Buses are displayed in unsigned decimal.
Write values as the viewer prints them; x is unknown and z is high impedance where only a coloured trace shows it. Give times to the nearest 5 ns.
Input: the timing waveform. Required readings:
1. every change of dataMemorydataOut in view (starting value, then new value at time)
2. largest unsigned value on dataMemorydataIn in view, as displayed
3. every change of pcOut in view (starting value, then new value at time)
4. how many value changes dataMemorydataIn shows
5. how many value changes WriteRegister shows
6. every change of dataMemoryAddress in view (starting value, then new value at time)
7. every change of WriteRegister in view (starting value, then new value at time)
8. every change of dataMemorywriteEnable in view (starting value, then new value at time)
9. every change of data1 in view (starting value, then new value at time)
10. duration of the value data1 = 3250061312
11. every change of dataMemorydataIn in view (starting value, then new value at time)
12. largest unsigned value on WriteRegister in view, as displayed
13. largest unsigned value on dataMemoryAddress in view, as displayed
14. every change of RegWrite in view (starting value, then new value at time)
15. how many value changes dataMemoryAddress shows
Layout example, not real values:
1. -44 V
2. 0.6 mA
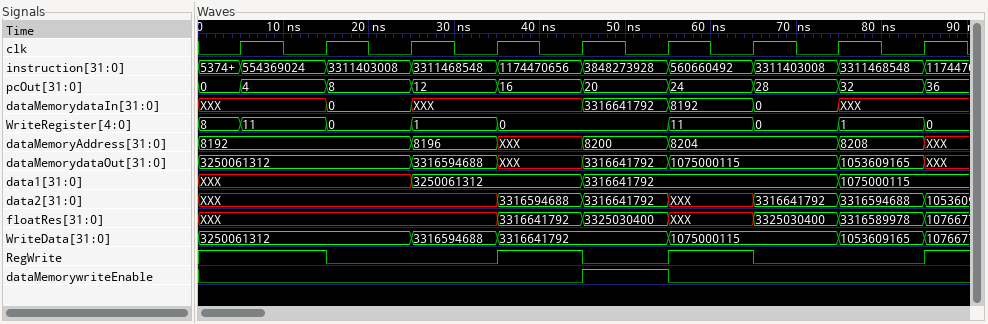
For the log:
1. 3250061312, 3316594688 at 25 ns, XXX at 35 ns, 3316641792 at 45 ns, 1075000115 at 55 ns, 1053609165 at 75 ns, XXX at 85 ns
2. 3316641792
3. 0, 4 at 5 ns, 8 at 15 ns, 12 at 25 ns, 16 at 35 ns, 20 at 45 ns, 24 at 55 ns, 28 at 65 ns, 32 at 75 ns, 36 at 85 ns
4. 6
5. 8
6. 8192, 8196 at 25 ns, XXX at 35 ns, 8200 at 45 ns, 8204 at 55 ns, 8208 at 75 ns, XXX at 85 ns
7. 8, 11 at 5 ns, 0 at 15 ns, 1 at 25 ns, 0 at 35 ns, 11 at 55 ns, 0 at 65 ns, 1 at 75 ns, 0 at 85 ns
8. 0, 1 at 45 ns, 0 at 55 ns
9. XXX, 3250061312 at 25 ns, 3316641792 at 45 ns, 1075000115 at 75 ns
10. 20 ns
11. XXX, 0 at 15 ns, XXX at 25 ns, 3316641792 at 45 ns, 8192 at 55 ns, 0 at 65 ns, XXX at 75 ns
12. 11
13. 8208
14. 1, 0 at 15 ns, 1 at 35 ns, 0 at 45 ns, 1 at 55 ns, 0 at 65 ns, 1 at 85 ns
15. 6
